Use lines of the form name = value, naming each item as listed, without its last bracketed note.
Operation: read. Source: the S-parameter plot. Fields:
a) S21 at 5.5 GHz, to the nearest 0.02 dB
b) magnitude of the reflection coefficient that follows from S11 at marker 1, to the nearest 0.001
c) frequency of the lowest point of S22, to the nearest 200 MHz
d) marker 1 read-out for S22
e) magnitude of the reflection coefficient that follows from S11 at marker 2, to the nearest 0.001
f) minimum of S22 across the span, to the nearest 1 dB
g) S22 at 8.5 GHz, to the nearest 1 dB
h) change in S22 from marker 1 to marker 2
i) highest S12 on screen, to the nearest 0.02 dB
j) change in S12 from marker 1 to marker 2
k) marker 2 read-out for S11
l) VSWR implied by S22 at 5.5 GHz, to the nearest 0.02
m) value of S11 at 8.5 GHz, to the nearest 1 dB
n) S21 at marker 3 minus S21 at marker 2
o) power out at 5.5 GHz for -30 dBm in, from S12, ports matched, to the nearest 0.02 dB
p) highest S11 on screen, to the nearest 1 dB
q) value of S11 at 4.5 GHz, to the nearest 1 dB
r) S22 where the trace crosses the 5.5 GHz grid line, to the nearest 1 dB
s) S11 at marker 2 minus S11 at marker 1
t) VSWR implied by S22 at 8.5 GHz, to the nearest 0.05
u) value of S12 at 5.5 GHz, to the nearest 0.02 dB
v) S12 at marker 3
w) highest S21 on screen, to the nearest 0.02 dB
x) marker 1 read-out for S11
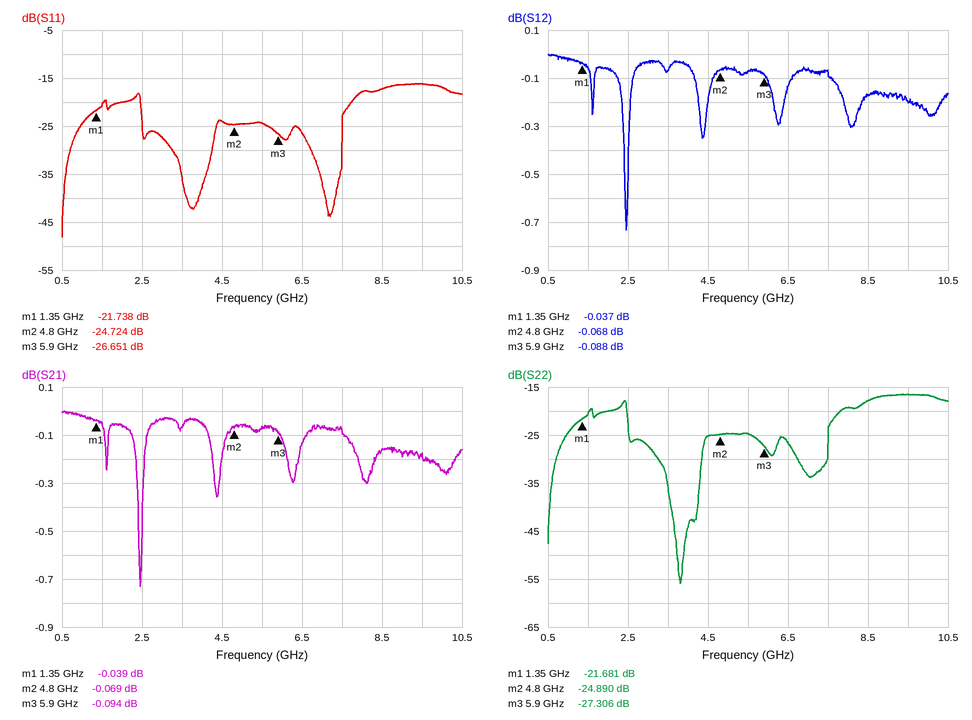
S21 at 5.5 GHz, to the nearest 0.02 dB = -0.06 dB
magnitude of the reflection coefficient that follows from S11 at marker 1, to the nearest 0.001 = 0.082
frequency of the lowest point of S22, to the nearest 200 MHz = 3.8 GHz
marker 1 read-out for S22 = -21.681 dB
magnitude of the reflection coefficient that follows from S11 at marker 2, to the nearest 0.001 = 0.058
minimum of S22 across the span, to the nearest 1 dB = -56 dB
S22 at 8.5 GHz, to the nearest 1 dB = -18 dB
change in S22 from marker 1 to marker 2 = -3.209 dB
highest S12 on screen, to the nearest 0.02 dB = 0.00 dB
change in S12 from marker 1 to marker 2 = -0.031 dB
marker 2 read-out for S11 = -24.724 dB
VSWR implied by S22 at 5.5 GHz, to the nearest 0.02 = 1.12
value of S11 at 8.5 GHz, to the nearest 1 dB = -17 dB
S21 at marker 3 minus S21 at marker 2 = -0.025 dB
power out at 5.5 GHz for -30 dBm in, from S12, ports matched, to the nearest 0.02 dB = -30.08 dBm
highest S11 on screen, to the nearest 1 dB = -16 dB
value of S11 at 4.5 GHz, to the nearest 1 dB = -24 dB
S22 where the trace crosses the 5.5 GHz grid line, to the nearest 1 dB = -25 dB
S11 at marker 2 minus S11 at marker 1 = -2.986 dB
VSWR implied by S22 at 8.5 GHz, to the nearest 0.05 = 1.30
value of S12 at 5.5 GHz, to the nearest 0.02 dB = -0.08 dB
S12 at marker 3 = -0.088 dB
highest S21 on screen, to the nearest 0.02 dB = 0.00 dB
marker 1 read-out for S11 = -21.738 dB
